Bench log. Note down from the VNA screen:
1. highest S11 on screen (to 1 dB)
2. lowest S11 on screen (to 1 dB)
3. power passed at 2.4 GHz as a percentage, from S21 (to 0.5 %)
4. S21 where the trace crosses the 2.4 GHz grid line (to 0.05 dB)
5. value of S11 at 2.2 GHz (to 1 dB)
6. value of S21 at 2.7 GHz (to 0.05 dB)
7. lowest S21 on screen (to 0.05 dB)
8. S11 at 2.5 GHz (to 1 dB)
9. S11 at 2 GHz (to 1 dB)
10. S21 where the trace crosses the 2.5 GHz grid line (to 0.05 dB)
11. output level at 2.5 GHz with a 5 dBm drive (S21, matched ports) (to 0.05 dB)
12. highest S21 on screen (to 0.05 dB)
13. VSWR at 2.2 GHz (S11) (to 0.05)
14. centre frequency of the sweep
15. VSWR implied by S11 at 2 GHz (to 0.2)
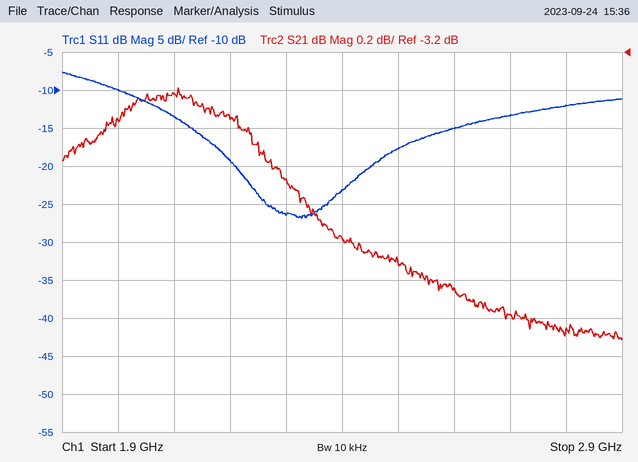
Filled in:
-8 dB
-27 dB
38.0 %
-4.20 dB
-19 dB
-4.60 dB
-4.70 dB
-18 dB
-10 dB
-4.30 dB
0.70 dBm
-3.40 dB
1.25
2.4 GHz
2.0
